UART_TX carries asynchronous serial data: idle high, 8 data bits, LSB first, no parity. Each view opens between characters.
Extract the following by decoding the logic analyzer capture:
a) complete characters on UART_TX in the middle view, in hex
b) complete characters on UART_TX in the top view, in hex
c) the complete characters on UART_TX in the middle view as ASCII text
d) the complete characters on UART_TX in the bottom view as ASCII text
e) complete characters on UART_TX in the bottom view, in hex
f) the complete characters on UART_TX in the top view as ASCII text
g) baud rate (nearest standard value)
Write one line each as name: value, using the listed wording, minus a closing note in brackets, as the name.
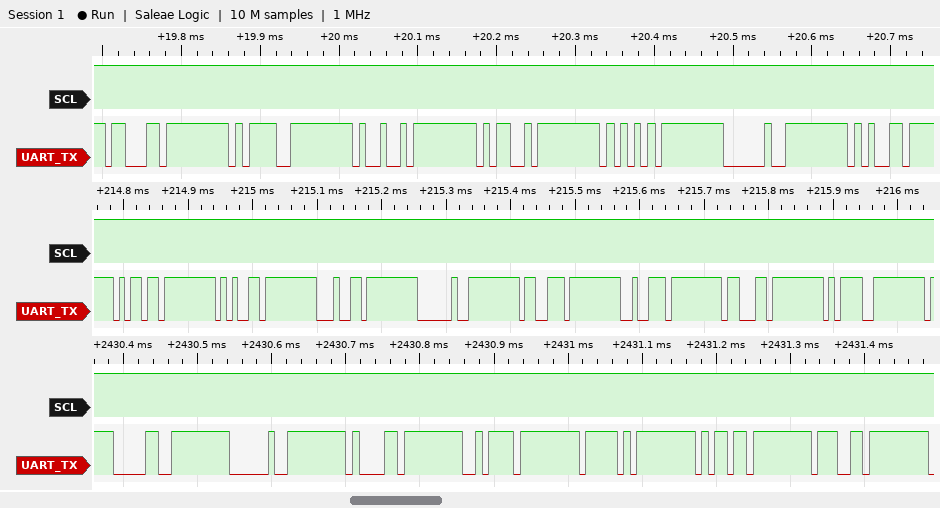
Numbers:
complete characters on UART_TX in the middle view, in hex: 6D, 65, 64, 20, 73, 72, 63, 3D
complete characters on UART_TX in the top view, in hex: 63, 3D, 49, 4D, 55, 20, 65
the complete characters on UART_TX in the middle view as ASCII text: "med src="
the complete characters on UART_TX in the bottom view as ASCII text: "0 az_mg"
complete characters on UART_TX in the bottom view, in hex: 30, 20, 61, 7A, 5F, 6D, 67
the complete characters on UART_TX in the top view as ASCII text: "c=IMU e"
baud rate: 115200 baud
